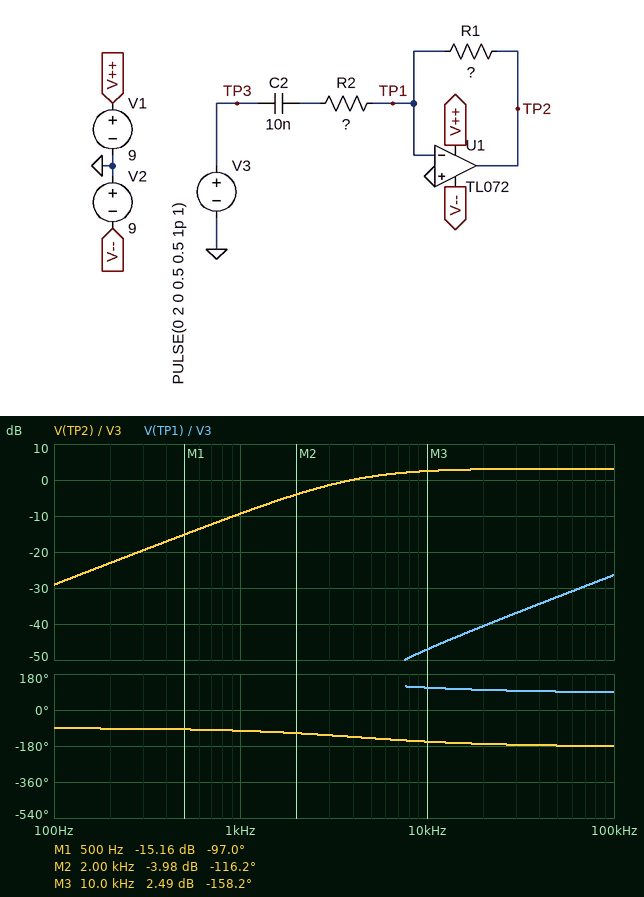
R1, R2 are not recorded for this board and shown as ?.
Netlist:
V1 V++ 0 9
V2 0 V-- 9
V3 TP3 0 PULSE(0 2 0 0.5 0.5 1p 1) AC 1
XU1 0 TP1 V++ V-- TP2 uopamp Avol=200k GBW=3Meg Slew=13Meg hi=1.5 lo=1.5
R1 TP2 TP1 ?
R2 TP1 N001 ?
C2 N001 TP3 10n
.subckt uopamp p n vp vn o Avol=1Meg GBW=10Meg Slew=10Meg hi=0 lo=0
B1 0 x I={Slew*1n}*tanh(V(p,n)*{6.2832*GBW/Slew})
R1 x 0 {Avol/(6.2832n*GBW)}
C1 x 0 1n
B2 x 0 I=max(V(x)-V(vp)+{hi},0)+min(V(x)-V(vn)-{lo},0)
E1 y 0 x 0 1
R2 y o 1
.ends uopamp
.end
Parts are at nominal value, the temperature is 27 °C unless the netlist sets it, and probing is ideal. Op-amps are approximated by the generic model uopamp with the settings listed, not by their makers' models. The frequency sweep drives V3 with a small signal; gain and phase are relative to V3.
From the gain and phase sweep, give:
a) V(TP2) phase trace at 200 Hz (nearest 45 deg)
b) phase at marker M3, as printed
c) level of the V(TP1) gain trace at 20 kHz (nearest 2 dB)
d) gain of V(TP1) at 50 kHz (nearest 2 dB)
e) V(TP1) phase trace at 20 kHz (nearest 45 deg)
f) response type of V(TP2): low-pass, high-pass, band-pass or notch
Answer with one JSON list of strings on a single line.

["-90 deg", "-158.2 deg", "-40 dB", "-32 dB", "90 deg", "high-pass"]
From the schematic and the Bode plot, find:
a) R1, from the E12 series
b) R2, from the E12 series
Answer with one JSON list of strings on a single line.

["5.6 kΩ", "3.9 kΩ"]
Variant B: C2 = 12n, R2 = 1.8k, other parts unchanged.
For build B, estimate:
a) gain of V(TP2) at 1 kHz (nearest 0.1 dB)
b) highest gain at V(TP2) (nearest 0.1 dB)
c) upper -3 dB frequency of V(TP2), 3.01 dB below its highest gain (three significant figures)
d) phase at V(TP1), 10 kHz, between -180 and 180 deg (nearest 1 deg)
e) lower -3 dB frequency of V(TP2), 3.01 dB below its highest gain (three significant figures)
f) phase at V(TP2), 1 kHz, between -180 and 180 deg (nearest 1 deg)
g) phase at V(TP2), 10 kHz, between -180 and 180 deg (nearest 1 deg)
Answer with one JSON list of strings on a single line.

["-7.6 dB", "9.8 dB", "739 kHz", "126 deg", "7.28 kHz", "-98 deg", "-144 deg"]
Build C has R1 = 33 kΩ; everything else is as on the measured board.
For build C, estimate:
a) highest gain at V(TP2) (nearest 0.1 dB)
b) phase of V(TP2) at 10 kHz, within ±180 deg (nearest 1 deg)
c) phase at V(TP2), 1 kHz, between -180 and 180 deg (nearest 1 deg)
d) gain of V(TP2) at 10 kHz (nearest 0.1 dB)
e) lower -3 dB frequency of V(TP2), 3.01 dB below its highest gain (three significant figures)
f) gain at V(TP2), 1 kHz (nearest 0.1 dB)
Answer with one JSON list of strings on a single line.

["18.5 dB", "-159 deg", "-104 deg", "18.0 dB", "4.02 kHz", "6.1 dB"]
